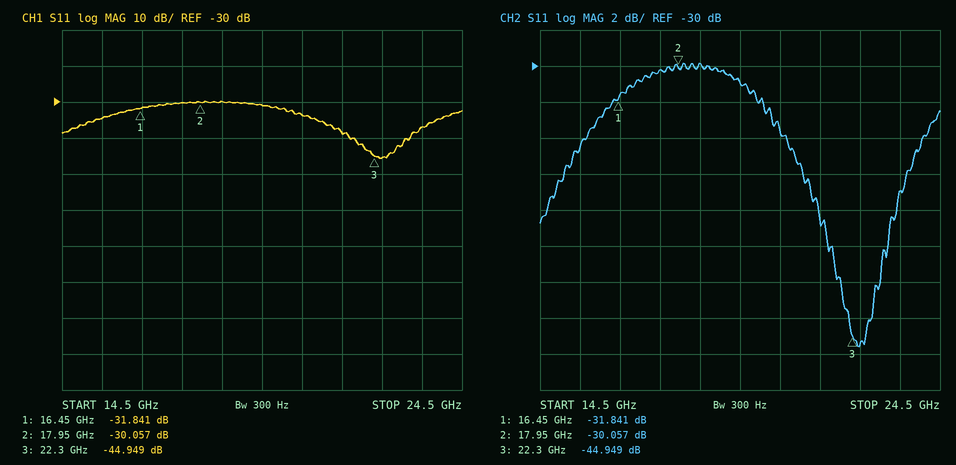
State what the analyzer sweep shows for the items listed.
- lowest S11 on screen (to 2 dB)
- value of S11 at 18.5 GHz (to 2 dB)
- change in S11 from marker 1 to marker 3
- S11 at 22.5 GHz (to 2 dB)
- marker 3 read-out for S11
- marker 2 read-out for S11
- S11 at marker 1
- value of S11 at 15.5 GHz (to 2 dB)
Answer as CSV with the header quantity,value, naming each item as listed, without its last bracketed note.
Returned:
quantity,value
lowest S11 on screen,-46 dB
value of S11 at 18.5 GHz,-30 dB
change in S11 from marker 1 to marker 3,-13.108 dB
S11 at 22.5 GHz,-46 dB
marker 3 read-out for S11,-44.949 dB
marker 2 read-out for S11,-30.057 dB
S11 at marker 1,-31.841 dB
value of S11 at 15.5 GHz,-34 dB
